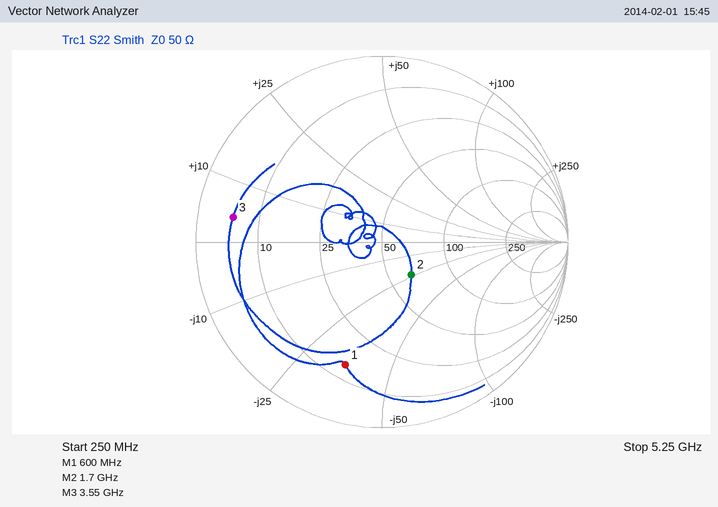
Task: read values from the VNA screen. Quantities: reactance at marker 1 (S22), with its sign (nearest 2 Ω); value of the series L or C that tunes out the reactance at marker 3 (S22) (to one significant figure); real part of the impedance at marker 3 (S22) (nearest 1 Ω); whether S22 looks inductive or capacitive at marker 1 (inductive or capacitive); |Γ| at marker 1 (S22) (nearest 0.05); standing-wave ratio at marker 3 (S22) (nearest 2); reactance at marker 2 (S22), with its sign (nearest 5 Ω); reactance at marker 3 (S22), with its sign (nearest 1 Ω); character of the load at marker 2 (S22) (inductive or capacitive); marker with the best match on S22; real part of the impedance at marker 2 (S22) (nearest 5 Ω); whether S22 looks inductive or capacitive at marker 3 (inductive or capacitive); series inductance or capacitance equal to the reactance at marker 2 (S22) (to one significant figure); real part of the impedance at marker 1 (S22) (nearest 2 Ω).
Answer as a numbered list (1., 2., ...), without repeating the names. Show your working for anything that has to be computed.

1. -36 Ω
2. C = 1/(2π × 3.55 GHz × 4 Ω) ≈ 11.2 pF, so 10 pF to one significant figure
3. 5 Ω
4. capacitive
5. 0.70
6. 10
7. -25 Ω
8. +4 Ω
9. capacitive
10. marker 2
11. 65 Ω
12. inductive
13. C = 1/(2π × 1.7 GHz × 25 Ω) ≈ 4 pF
14. 14 Ω
